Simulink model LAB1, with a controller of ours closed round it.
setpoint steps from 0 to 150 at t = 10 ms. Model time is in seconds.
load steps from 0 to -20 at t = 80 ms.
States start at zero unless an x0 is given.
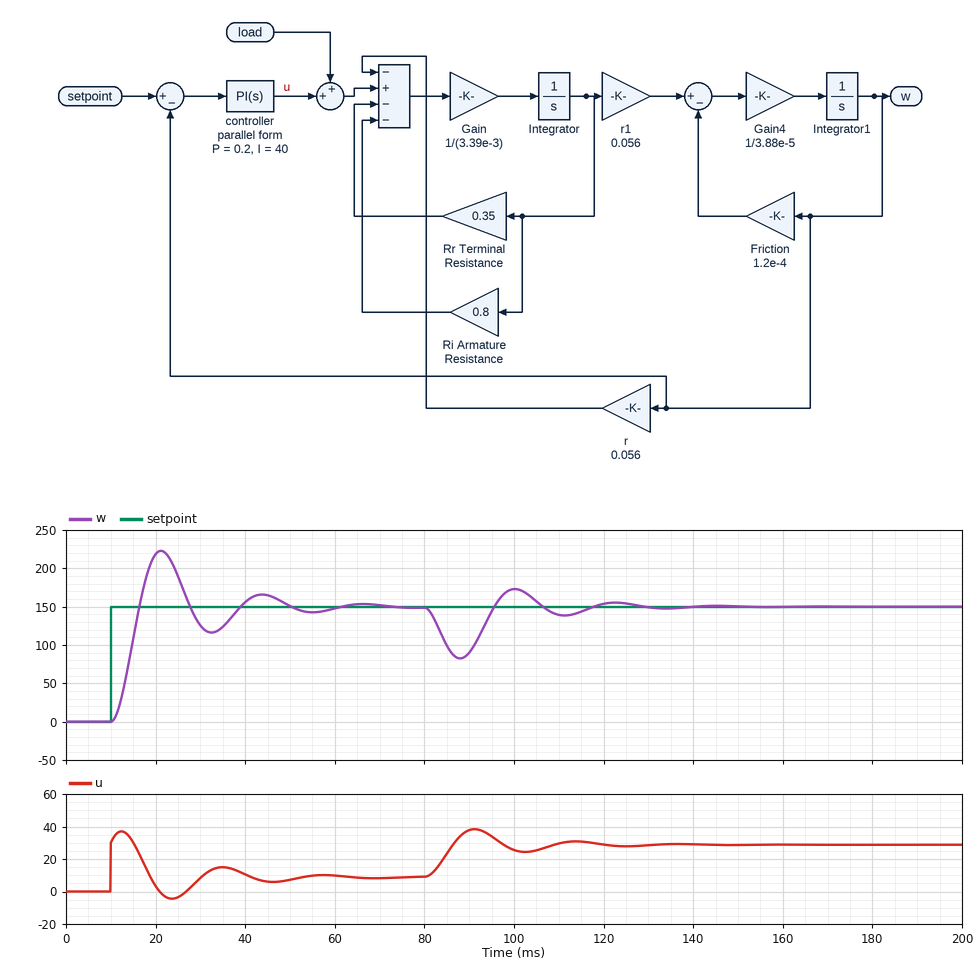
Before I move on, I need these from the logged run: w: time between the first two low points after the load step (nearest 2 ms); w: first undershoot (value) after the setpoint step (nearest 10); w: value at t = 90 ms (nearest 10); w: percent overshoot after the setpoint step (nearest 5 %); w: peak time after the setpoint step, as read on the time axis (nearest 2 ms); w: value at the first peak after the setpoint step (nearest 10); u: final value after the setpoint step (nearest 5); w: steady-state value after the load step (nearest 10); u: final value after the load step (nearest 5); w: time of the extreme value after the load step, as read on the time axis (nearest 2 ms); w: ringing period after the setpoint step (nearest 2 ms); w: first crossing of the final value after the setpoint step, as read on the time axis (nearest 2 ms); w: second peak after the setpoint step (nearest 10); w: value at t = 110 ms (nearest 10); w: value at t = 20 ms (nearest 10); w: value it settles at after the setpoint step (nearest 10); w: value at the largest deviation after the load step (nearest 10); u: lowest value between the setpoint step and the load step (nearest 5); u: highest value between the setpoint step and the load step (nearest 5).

24 ms
120
90
50 %
22 ms
220
10
150
30
88 ms
22 ms
16 ms
170
140
220
150
80
-5
35
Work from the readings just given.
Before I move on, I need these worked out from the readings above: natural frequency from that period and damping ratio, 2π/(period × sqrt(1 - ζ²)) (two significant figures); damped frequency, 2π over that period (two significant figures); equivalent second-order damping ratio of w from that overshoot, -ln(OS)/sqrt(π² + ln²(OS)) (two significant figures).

0.29 rad/ms
0.29 rad/ms
0.22
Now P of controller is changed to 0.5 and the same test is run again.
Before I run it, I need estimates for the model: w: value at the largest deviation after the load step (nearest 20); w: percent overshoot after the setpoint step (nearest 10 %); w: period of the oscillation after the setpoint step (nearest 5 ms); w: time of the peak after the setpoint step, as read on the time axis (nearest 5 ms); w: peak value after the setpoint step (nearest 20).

100
40 %
15 ms
15 ms
200
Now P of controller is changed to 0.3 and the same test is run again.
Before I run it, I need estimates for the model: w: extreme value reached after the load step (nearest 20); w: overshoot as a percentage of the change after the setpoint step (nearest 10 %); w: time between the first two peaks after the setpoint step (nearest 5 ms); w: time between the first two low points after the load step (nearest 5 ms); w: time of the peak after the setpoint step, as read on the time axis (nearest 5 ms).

100
40 %
20 ms
20 ms
20 ms
